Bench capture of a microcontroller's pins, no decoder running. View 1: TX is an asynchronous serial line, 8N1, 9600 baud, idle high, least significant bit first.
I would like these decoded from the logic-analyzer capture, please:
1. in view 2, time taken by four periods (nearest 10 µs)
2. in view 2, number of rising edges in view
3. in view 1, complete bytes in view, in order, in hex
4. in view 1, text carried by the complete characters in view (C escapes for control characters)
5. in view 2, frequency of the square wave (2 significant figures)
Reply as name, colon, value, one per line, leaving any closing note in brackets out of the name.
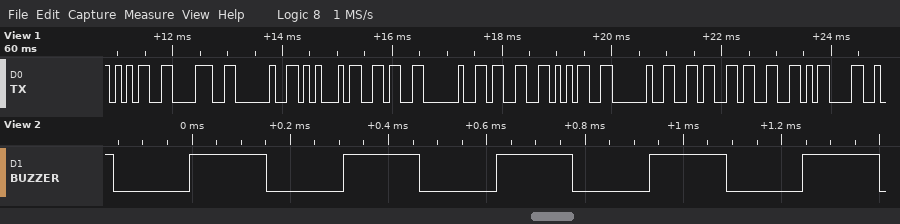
in view 2, time taken by four periods: 1250 µs
in view 2, number of rising edges in view: 5
in view 1, complete bytes in view, in order, in hex: 35 38 20 45 36 20 33 35 20 36 33 0D
in view 1, text carried by the complete characters in view: "58 E6 35 63\r"
in view 2, frequency of the square wave: 3.2 kHz
